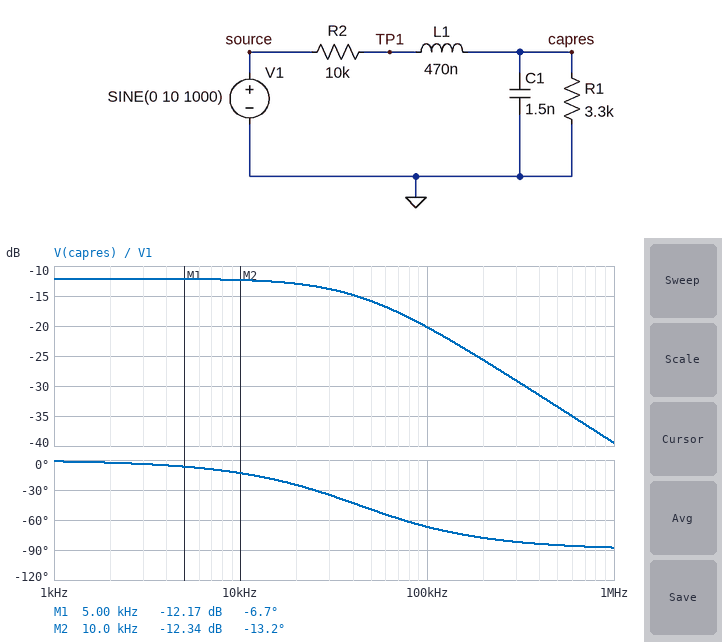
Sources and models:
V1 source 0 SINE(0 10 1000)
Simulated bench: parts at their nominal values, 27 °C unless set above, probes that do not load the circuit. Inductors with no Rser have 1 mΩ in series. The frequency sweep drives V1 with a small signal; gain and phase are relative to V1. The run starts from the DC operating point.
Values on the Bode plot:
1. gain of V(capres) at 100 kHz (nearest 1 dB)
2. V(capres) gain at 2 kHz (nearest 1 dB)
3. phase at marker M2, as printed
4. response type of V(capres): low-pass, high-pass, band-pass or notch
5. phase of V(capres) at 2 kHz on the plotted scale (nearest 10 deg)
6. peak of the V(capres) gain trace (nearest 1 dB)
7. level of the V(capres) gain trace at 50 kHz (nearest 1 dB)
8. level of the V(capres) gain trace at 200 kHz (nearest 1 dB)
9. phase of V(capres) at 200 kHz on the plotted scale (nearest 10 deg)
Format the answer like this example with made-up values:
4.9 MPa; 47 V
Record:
-20 dB; -12 dB; -13.2 deg; low-pass; 0 deg; -12 dB; -16 dB; -26 dB; -80 deg
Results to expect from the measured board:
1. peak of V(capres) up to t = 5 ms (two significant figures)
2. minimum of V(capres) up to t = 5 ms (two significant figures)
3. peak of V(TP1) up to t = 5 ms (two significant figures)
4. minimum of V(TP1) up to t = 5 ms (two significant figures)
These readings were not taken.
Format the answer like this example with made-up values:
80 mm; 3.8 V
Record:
2.5 V; -2.5 V; 2.5 V; -2.5 V
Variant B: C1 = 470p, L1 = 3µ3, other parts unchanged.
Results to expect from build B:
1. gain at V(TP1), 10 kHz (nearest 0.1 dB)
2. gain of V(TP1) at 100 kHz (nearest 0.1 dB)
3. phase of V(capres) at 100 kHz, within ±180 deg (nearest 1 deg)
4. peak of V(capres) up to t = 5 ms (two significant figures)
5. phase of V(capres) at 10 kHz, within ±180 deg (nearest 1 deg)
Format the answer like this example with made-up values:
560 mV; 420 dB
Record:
-12.1 dB; -14.0 dB; -36 deg; 2.5 V; -4 deg
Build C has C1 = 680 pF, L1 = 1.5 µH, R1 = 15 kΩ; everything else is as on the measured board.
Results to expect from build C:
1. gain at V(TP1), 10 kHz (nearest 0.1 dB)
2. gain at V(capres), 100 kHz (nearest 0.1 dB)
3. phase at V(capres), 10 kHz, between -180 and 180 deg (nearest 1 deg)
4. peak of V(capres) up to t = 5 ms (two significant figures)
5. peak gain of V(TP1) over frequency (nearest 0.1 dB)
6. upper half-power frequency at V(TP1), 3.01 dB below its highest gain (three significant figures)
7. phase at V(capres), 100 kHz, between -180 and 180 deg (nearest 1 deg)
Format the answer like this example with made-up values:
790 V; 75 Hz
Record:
-4.7 dB; -13.2 dB; -14 deg; 6.0 V; -4.4 dB; 39.0 kHz; -69 deg
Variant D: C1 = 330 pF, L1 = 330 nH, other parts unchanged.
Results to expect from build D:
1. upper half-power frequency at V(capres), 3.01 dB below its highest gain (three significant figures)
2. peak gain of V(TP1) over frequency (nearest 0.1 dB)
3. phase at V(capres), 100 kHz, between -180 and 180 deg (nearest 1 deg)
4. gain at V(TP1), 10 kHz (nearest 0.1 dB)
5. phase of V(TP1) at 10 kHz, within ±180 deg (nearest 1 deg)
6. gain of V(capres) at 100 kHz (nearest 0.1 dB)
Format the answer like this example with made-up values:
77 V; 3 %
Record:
194 kHz; -12.1 dB; -27 deg; -12.1 dB; -3 deg; -13.1 dB
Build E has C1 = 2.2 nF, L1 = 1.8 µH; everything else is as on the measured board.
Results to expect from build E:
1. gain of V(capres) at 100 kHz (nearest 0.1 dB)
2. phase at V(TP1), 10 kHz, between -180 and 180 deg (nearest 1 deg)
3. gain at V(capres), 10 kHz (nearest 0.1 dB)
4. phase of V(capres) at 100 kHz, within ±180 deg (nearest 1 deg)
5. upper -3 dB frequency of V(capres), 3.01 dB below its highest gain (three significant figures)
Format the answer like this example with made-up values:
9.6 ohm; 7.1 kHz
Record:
-23.2 dB; -19 deg; -12.6 dB; -74 deg; 29.2 kHz
